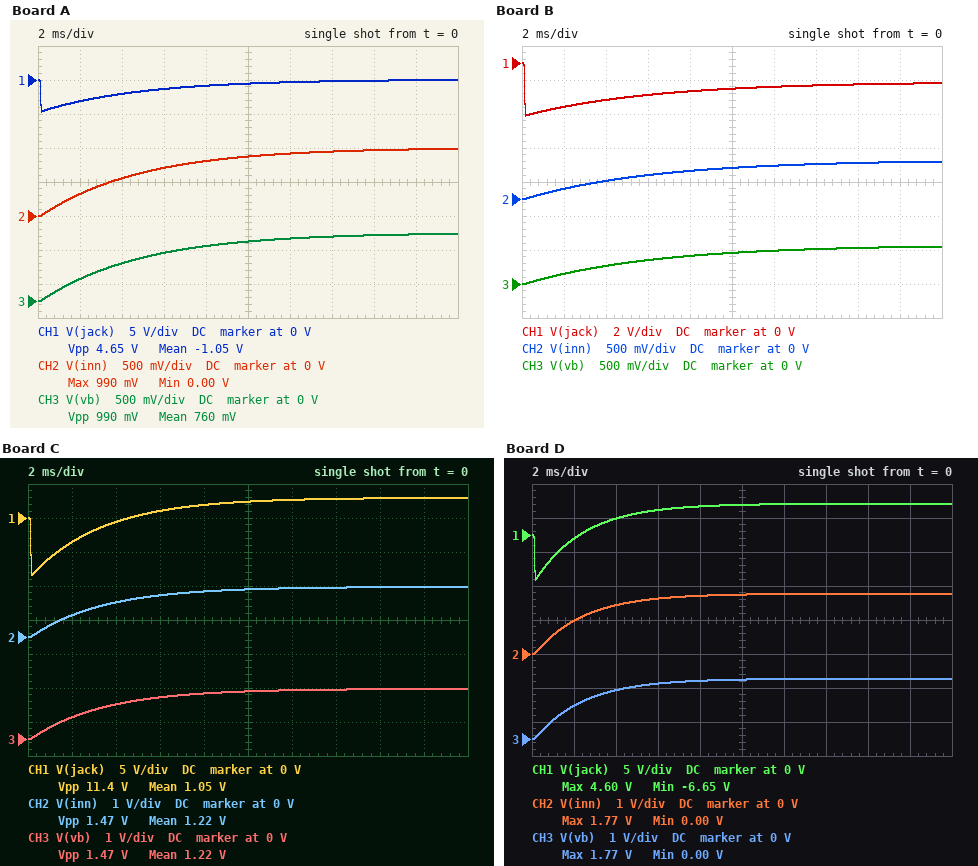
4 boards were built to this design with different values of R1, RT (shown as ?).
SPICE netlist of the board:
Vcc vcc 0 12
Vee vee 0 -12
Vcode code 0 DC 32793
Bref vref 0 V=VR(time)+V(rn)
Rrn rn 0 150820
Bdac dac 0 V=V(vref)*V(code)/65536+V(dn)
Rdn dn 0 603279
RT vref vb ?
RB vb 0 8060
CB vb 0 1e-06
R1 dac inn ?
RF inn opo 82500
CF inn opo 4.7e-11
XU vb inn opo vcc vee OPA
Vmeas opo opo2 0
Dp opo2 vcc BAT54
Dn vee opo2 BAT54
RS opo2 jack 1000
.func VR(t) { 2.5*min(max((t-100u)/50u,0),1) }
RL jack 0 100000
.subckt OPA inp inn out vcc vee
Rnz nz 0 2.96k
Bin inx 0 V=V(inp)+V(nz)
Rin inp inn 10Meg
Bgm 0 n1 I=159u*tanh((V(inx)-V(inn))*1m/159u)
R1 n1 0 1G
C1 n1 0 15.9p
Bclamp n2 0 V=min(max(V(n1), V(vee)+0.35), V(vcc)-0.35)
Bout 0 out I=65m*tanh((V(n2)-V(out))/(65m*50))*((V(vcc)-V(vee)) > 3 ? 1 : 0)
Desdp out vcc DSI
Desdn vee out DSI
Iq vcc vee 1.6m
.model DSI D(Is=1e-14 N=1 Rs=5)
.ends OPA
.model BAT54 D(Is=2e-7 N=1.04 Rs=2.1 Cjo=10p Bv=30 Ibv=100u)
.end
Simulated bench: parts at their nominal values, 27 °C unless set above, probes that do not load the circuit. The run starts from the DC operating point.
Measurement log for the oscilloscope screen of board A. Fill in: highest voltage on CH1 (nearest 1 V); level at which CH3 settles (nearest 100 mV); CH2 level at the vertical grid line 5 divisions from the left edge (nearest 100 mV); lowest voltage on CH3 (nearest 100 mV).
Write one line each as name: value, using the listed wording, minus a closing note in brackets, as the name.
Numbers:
highest voltage on CH1: 0 V
level at which CH3 settles: 1.0 V
CH2 level at the vertical grid line 5 divisions from the left edge: 900 mV
lowest voltage on CH3: 0 V
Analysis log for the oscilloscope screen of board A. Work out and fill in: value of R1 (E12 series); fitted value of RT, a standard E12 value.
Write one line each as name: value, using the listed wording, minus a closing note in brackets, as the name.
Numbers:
value of R1: 22 kΩ
fitted value of RT, a standard E12 value: 12 kΩ
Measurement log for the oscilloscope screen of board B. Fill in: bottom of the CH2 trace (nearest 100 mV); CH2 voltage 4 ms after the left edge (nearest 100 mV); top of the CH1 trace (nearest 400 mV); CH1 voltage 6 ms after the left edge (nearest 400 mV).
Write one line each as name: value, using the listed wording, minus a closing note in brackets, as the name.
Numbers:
bottom of the CH2 trace: 0 V
CH2 voltage 4 ms after the left edge: 300 mV
top of the CH1 trace: 0 V
CH1 voltage 6 ms after the left edge: -2.0 V
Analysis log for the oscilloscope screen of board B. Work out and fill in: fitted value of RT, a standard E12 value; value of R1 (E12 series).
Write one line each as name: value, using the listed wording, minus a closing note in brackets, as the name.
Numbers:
fitted value of RT, a standard E12 value: 27 kΩ
value of R1: 33 kΩ
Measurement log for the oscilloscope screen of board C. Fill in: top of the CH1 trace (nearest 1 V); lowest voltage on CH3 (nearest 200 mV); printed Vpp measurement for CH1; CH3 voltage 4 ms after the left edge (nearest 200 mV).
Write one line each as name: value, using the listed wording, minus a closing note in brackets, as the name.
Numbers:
top of the CH1 trace: 3 V
lowest voltage on CH3: 0 V
printed Vpp measurement for CH1: 11.4 V
CH3 voltage 4 ms after the left edge: 1.0 V
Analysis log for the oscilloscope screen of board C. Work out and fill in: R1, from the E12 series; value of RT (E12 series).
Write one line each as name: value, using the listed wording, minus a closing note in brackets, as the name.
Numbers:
R1, from the E12 series: 12 kΩ
value of RT: 5.6 kΩ
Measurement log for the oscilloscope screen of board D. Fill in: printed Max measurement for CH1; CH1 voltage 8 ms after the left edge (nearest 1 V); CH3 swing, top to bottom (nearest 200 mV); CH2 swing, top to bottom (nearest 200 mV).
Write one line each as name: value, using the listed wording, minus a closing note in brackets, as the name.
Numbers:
printed Max measurement for CH1: 4.60 V
CH1 voltage 8 ms after the left edge: 4 V
CH3 swing, top to bottom: 1.8 V
CH2 swing, top to bottom: 1.8 V
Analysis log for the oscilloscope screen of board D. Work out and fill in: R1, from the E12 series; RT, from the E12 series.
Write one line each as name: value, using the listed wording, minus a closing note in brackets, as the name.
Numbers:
R1, from the E12 series: 15 kΩ
RT, from the E12 series: 3.3 kΩ
